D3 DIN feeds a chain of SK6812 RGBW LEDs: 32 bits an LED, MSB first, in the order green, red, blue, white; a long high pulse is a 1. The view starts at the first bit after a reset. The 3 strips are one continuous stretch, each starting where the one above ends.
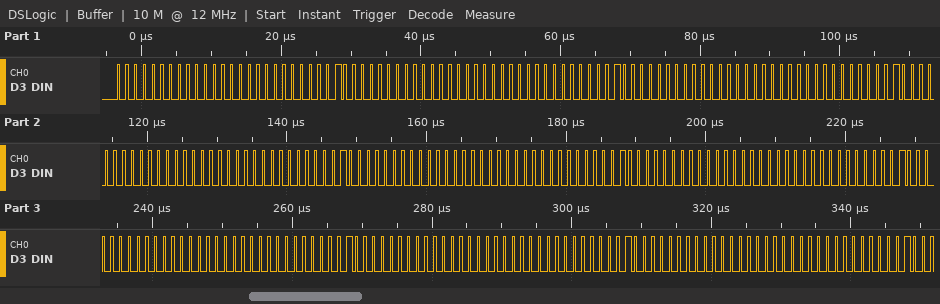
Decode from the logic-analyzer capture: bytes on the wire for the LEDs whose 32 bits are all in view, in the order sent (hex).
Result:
00 00 00 40 00 00 00 40 00 00 00 40 00 00 00 40 00 00 00 40 00 00 00 40 00 00 00 40 00 00 00 40
